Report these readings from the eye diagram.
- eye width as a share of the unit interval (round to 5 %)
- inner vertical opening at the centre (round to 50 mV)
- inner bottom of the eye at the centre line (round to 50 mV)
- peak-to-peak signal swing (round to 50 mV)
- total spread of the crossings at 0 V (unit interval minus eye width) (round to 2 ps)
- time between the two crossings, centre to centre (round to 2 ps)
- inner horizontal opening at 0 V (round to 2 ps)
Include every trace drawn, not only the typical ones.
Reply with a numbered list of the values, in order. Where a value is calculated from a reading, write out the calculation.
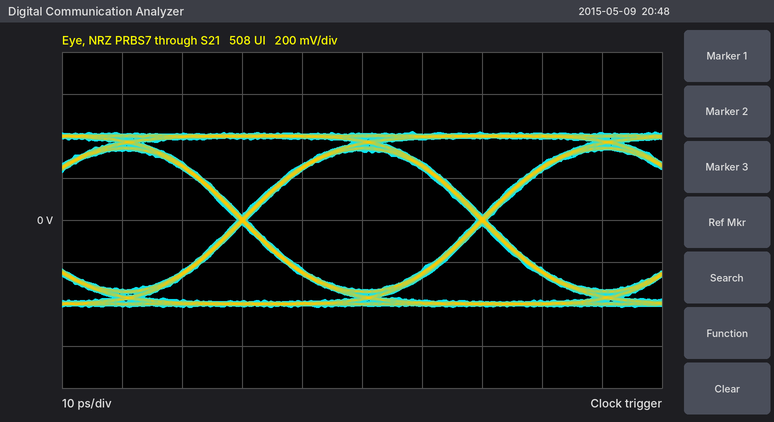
1. 38 ps / 40 ps ≈ 95 %
2. 650 mV
3. -350 mV
4. 850 mV
5. 2 ps
6. 40 ps
7. 38 ps
